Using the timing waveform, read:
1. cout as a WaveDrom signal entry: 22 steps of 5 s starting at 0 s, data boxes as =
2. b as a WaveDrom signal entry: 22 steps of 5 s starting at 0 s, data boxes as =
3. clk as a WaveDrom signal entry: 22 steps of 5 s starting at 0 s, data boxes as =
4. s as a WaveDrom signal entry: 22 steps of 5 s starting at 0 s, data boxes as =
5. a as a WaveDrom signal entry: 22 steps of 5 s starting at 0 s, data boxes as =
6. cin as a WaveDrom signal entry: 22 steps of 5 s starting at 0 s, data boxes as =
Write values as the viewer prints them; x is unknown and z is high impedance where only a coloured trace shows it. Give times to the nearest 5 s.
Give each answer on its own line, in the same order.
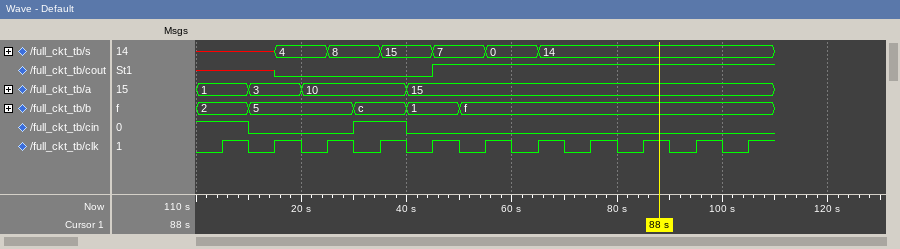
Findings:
{name: 'cout', wave: 'x..0.....1............'}
{name: 'b', wave: '=.=...=.=.=...........', data: '2 5 c 1 f'}
{name: 'clk', wave: '0101010101010101010101'}
{name: 's', wave: 'x..=.=.=.=.=.=........', data: '4 8 15 7 0 14'}
{name: 'a', wave: '=.=.=...=.............', data: '1 3 10 15'}
{name: 'cin', wave: '1.0...1.0.............'}
